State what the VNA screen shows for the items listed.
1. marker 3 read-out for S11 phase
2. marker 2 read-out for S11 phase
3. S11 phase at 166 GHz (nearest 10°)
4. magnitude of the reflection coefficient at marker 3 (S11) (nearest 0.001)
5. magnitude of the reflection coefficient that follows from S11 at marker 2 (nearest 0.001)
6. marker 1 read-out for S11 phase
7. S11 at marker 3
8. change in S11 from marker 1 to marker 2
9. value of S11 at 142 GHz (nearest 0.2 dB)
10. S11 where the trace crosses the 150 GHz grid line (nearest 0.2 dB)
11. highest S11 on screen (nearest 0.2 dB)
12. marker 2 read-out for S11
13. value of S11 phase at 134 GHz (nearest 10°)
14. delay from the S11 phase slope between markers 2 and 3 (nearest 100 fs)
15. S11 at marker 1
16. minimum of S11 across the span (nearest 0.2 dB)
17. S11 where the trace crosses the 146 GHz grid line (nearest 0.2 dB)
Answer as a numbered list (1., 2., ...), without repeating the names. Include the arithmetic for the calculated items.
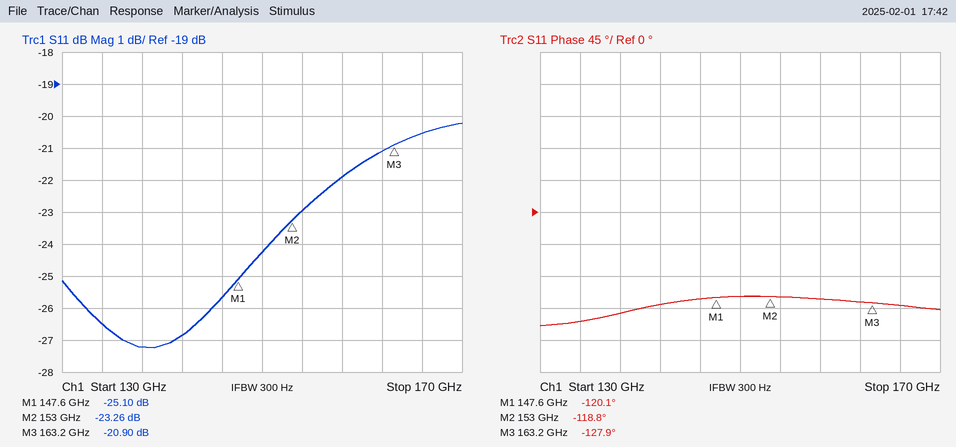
1. -127.9°
2. -118.8°
3. -130°
4. 10^(-20.9/20) ≈ 0.090
5. 10^(-23.26/20) ≈ 0.069
6. -120.1°
7. -20.90 dB
8. -23.26 − (-25.1) = 1.84 dB
9. -26.8 dB
10. -24.2 dB
11. -20.2 dB
12. -23.26 dB
13. -150°
14. −(-127.9° − (-118.8°))/(360° × 10.2 GHz) ≈ 2.5 ps
15. -25.10 dB
16. -27.2 dB
17. -25.6 dB
